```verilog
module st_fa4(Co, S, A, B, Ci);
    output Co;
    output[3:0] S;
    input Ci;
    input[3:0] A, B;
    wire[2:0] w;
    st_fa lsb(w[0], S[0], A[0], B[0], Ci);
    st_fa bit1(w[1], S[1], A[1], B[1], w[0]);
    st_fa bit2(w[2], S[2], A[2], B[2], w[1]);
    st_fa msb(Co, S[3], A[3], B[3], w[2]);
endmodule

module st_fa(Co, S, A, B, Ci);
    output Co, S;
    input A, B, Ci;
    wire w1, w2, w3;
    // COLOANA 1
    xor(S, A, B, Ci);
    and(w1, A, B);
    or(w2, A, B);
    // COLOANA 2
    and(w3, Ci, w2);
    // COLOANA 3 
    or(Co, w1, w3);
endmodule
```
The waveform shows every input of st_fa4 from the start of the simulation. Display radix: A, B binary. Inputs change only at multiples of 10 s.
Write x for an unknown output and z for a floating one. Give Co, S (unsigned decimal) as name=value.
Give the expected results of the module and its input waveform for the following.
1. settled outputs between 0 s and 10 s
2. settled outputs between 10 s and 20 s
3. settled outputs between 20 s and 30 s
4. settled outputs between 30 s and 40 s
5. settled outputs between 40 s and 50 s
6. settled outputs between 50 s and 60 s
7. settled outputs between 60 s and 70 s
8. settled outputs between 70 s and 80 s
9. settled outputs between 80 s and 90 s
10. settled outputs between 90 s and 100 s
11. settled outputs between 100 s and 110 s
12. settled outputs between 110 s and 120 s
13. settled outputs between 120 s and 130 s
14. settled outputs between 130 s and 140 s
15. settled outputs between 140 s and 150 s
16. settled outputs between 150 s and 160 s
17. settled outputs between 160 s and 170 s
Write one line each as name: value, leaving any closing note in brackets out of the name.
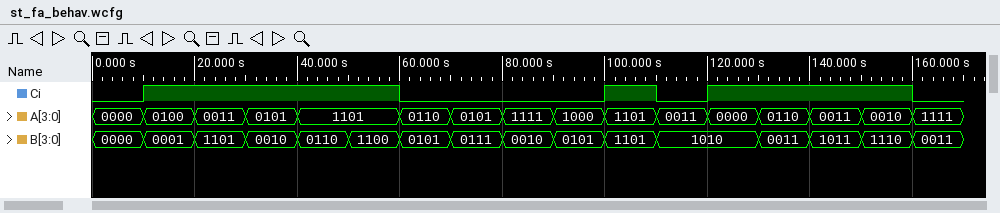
settled outputs between 0 s and 10 s: Co=0, S=0
settled outputs between 10 s and 20 s: Co=0, S=6
settled outputs between 20 s and 30 s: Co=1, S=1
settled outputs between 30 s and 40 s: Co=0, S=8
settled outputs between 40 s and 50 s: Co=1, S=4
settled outputs between 50 s and 60 s: Co=1, S=10
settled outputs between 60 s and 70 s: Co=0, S=11
settled outputs between 70 s and 80 s: Co=0, S=12
settled outputs between 80 s and 90 s: Co=1, S=1
settled outputs between 90 s and 100 s: Co=0, S=13
settled outputs between 100 s and 110 s: Co=1, S=11
settled outputs between 110 s and 120 s: Co=0, S=13
settled outputs between 120 s and 130 s: Co=0, S=11
settled outputs between 130 s and 140 s: Co=0, S=10
settled outputs between 140 s and 150 s: Co=0, S=15
settled outputs between 150 s and 160 s: Co=1, S=1
settled outputs between 160 s and 170 s: Co=1, S=2
